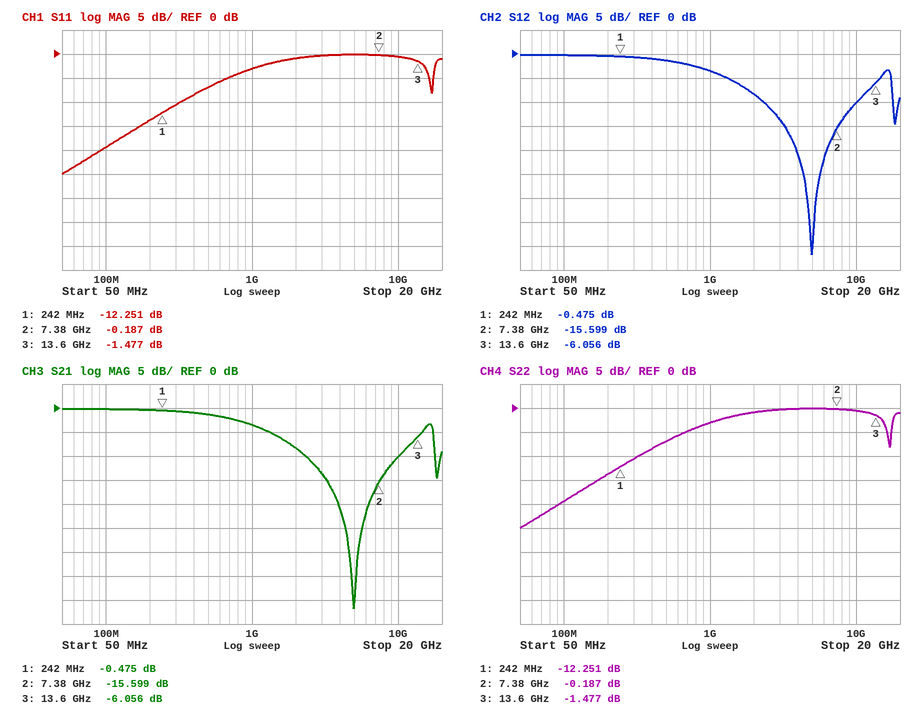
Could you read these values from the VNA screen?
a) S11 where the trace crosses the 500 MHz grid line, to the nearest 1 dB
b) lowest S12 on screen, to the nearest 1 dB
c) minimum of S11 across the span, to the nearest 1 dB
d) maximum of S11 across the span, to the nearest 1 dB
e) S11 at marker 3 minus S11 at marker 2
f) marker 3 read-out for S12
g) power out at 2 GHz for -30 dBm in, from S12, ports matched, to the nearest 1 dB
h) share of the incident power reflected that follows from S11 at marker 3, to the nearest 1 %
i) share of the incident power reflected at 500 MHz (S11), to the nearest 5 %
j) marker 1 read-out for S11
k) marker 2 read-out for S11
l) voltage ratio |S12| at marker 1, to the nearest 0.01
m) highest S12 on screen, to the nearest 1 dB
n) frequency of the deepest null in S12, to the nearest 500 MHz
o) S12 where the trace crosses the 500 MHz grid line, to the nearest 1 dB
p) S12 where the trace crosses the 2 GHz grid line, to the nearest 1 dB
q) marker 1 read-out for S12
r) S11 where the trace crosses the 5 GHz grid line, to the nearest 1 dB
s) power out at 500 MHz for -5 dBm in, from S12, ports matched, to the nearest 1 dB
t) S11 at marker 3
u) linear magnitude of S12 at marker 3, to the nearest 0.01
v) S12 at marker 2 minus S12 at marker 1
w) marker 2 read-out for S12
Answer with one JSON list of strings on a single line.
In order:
["-7 dB", "-42 dB", "-25 dB", "0 dB", "-1.290 dB", "-6.056 dB", "-38 dBm", "71 %", "20 %", "-12.251 dB", "-0.187 dB", "0.95", "0 dB", "5.0 GHz", "-1 dB", "-8 dB", "-0.475 dB", "0 dB", "-6 dBm", "-1.477 dB", "0.50", "-15.124 dB", "-15.599 dB"]
